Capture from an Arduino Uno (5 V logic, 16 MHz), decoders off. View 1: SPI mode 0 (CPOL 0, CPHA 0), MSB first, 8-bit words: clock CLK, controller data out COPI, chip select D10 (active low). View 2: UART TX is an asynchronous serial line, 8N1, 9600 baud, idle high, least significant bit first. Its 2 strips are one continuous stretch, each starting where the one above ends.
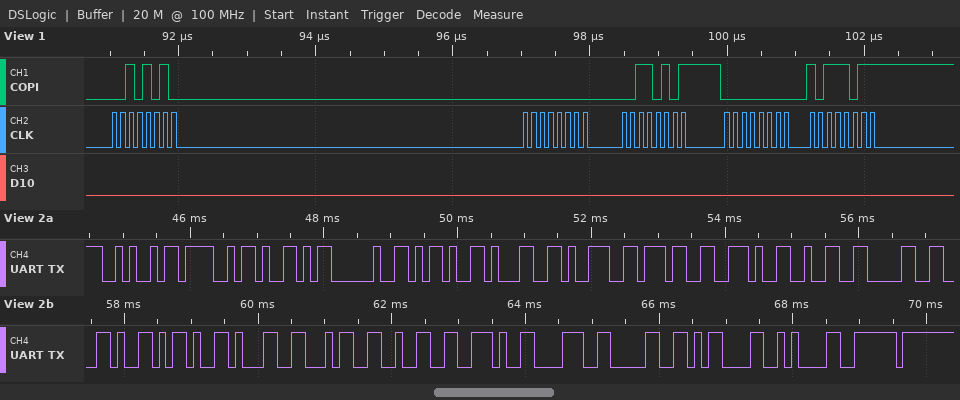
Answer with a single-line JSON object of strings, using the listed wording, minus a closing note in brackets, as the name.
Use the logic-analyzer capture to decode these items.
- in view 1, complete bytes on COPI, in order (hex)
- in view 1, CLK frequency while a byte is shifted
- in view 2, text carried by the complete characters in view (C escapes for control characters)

{"in view 1, complete bytes on COPI, in order": "0x2A 0x00 0x35 0x00 0xBB", "in view 1, CLK frequency while a byte is shifted": "8 MHz", "in view 2, text carried by the complete characters in view": "\"JOY -197.20,-142.80\\r\\n~\""}
